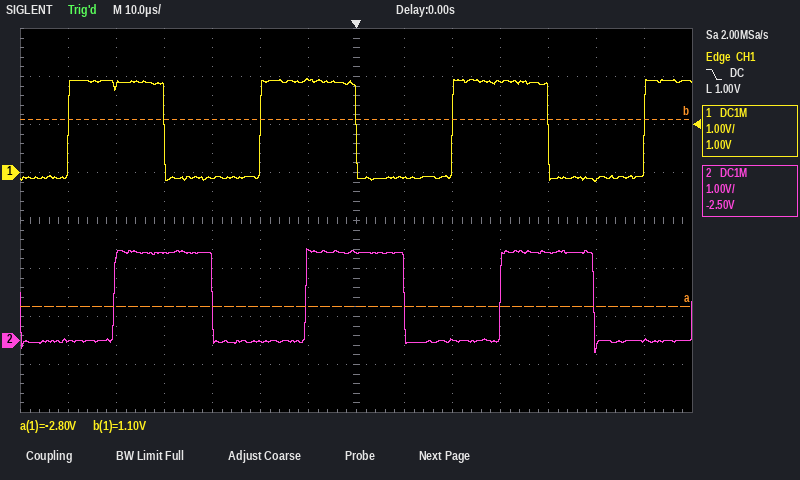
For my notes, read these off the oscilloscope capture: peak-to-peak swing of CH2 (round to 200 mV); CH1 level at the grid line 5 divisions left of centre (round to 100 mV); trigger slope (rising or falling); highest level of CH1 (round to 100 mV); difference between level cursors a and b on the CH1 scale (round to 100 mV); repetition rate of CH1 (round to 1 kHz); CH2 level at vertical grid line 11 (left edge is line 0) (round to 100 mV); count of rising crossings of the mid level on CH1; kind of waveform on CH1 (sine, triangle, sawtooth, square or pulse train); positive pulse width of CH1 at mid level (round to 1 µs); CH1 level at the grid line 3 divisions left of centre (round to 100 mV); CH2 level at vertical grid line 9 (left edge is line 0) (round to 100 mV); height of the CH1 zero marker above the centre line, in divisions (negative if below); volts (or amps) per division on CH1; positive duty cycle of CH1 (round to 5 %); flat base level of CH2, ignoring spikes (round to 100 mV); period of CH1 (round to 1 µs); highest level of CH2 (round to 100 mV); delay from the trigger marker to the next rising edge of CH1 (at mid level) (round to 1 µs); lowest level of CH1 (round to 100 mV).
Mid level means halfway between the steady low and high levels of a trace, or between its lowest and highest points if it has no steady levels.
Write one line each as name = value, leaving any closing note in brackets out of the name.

peak-to-peak swing of CH2 = 2.2 V
CH1 level at the grid line 5 divisions left of centre = 1.8 V
trigger slope = falling
highest level of CH1 = 2.0 V
difference between level cursors a and b on the CH1 scale = 3.9 V
repetition rate of CH1 = 25 kHz
CH2 level at vertical grid line 11 (left edge is line 0) = 1.8 V
count of rising crossings of the mid level on CH1 = 4
kind of waveform on CH1 = square
positive pulse width of CH1 at mid level = 20 µs
CH1 level at the grid line 3 divisions left of centre = -100 mV
CH2 level at vertical grid line 9 (left edge is line 0) = 0.0 V
height of the CH1 zero marker above the centre line, in divisions = +1.0 div
volts (or amps) per division on CH1 = 1 V
positive duty cycle of CH1 = 50 %
flat base level of CH2, ignoring spikes = 0.0 V
period of CH1 = 40 µs
highest level of CH2 = 1.9 V
delay from the trigger marker to the next rising edge of CH1 (at mid level) = 20 µs
lowest level of CH1 = -200 mV
